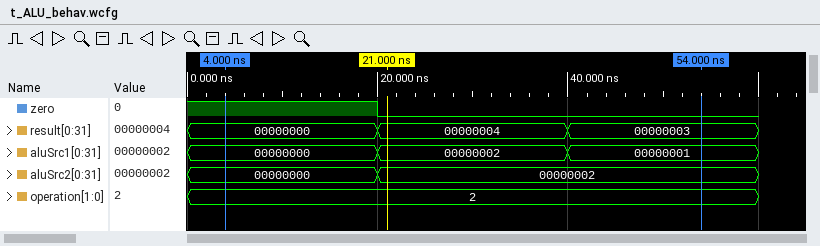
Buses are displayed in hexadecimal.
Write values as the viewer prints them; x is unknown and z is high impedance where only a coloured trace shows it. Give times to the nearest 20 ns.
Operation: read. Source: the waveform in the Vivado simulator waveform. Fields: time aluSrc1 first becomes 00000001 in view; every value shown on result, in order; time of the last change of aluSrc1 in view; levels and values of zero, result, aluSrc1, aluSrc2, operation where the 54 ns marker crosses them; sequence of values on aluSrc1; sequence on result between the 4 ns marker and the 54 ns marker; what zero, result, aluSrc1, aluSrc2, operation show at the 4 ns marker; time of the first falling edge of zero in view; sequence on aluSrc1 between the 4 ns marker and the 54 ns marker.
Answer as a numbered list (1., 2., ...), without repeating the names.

1. 40 ns
2. 00000000, 00000004, 00000003
3. 40 ns
4. zero=0, result=00000003, aluSrc1=00000001, aluSrc2=00000002, operation=2
5. 00000000, 00000002, 00000001
6. 00000000, 00000004, 00000003
7. zero=1, result=00000000, aluSrc1=00000000, aluSrc2=00000000, operation=2
8. 20 ns
9. 00000000, 00000002, 00000001
